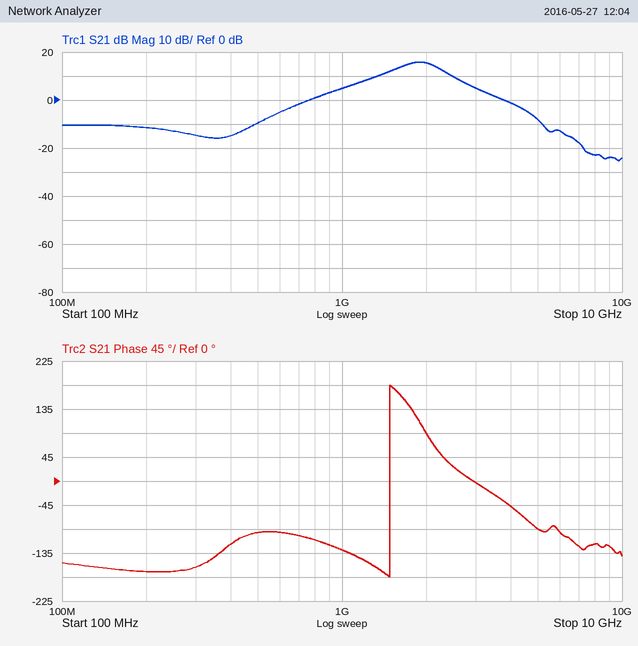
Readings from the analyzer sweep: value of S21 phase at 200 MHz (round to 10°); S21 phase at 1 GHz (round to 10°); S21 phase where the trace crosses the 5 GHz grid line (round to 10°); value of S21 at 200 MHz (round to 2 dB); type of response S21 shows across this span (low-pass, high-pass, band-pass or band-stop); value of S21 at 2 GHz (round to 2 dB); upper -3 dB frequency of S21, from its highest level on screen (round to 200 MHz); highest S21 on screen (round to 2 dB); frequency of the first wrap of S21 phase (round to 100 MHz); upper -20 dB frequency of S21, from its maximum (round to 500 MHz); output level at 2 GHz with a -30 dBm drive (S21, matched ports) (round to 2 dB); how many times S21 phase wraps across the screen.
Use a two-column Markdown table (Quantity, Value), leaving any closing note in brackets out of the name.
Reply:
| Quantity | Value |
|---|---|
| value of S21 phase at 200 MHz | -170° |
| S21 phase at 1 GHz | -130° |
| S21 phase where the trace crosses the 5 GHz grid line | -90° |
| value of S21 at 200 MHz | -12 dB |
| type of response S21 shows across this span | band-pass |
| value of S21 at 2 GHz | 16 dB |
| upper -3 dB frequency of S21, from its highest level on screen | 2.2 GHz |
| highest S21 on screen | 16 dB |
| frequency of the first wrap of S21 phase | 1.5 GHz |
| upper -20 dB frequency of S21, from its maximum | 4.5 GHz |
| output level at 2 GHz with a -30 dBm drive (S21, matched ports) | -14 dBm |
| how many times S21 phase wraps across the screen | 1 |
